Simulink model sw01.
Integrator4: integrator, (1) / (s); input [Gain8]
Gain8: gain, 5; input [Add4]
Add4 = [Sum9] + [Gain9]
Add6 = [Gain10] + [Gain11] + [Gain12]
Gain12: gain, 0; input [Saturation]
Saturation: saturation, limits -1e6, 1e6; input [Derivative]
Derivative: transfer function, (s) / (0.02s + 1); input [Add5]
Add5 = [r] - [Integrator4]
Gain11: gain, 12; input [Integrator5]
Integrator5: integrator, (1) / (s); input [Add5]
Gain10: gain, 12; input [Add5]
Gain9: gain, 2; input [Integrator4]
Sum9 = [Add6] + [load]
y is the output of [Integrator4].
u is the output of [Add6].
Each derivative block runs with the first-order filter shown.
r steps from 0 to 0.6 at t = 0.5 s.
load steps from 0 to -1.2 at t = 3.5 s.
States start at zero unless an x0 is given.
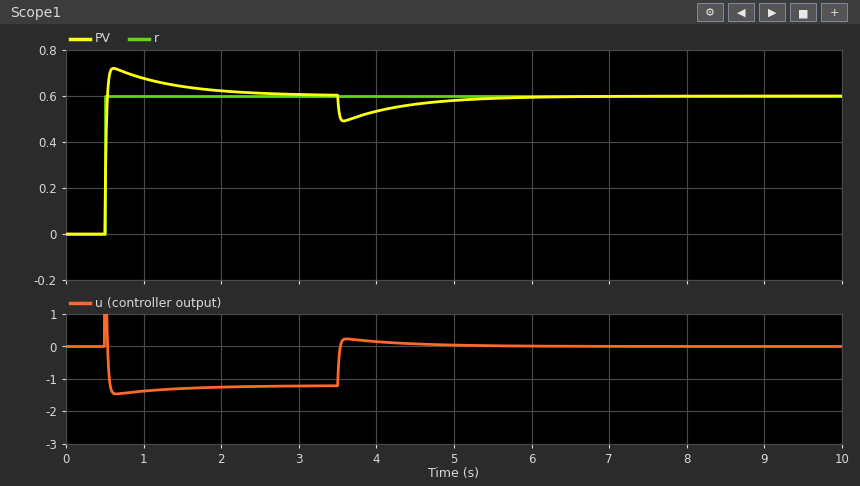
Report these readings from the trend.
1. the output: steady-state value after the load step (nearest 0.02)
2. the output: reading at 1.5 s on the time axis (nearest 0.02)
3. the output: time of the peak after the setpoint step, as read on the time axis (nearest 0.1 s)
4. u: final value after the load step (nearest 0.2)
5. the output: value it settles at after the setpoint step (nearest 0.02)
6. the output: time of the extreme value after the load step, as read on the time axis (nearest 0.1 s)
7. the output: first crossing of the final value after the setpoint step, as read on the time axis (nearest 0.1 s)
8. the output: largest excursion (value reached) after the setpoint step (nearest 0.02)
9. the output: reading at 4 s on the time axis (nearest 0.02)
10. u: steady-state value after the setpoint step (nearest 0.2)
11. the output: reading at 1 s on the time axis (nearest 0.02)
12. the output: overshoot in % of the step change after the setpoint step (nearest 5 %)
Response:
0.60
0.64
0.6 s
0.0
0.60
3.6 s
0.5 s
0.72
0.54
-1.2
0.68
20 %
